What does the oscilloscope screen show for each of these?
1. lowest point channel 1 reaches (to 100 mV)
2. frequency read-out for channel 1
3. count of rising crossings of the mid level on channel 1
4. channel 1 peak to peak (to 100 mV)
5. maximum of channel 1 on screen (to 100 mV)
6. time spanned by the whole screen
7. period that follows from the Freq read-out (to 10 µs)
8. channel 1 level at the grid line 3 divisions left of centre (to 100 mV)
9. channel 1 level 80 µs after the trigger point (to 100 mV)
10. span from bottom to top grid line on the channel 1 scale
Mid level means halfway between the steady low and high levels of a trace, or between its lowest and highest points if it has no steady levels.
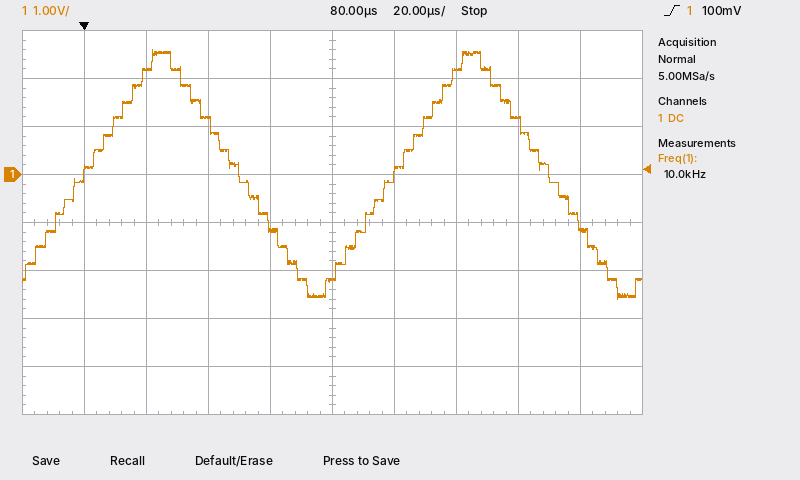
-2.6 V
10.0 kHz
2
5.2 V
2.6 V
200 µs
100 µs
2.2 V
-2.2 V
8 V
